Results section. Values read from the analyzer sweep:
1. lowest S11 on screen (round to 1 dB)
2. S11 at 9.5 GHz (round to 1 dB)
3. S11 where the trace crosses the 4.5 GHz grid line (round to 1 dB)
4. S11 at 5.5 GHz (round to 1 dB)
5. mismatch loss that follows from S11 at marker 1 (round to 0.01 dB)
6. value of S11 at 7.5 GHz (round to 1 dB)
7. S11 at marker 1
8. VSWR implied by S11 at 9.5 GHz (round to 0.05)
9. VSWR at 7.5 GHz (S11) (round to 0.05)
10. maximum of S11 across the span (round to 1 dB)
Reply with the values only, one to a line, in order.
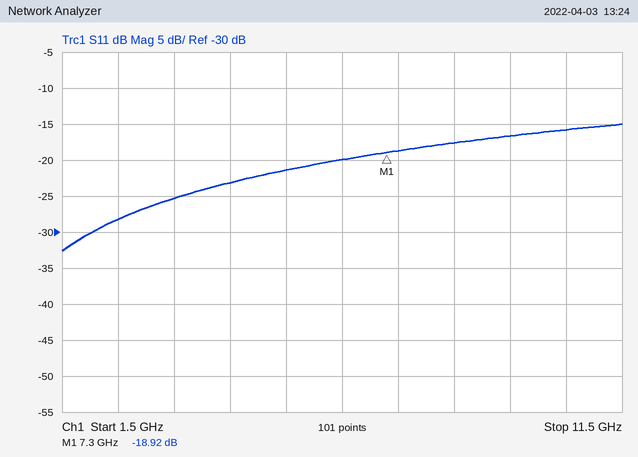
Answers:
-33 dB
-17 dB
-23 dB
-21 dB
0.06 dB
-19 dB
-18.92 dB
1.35
1.25
-15 dB
